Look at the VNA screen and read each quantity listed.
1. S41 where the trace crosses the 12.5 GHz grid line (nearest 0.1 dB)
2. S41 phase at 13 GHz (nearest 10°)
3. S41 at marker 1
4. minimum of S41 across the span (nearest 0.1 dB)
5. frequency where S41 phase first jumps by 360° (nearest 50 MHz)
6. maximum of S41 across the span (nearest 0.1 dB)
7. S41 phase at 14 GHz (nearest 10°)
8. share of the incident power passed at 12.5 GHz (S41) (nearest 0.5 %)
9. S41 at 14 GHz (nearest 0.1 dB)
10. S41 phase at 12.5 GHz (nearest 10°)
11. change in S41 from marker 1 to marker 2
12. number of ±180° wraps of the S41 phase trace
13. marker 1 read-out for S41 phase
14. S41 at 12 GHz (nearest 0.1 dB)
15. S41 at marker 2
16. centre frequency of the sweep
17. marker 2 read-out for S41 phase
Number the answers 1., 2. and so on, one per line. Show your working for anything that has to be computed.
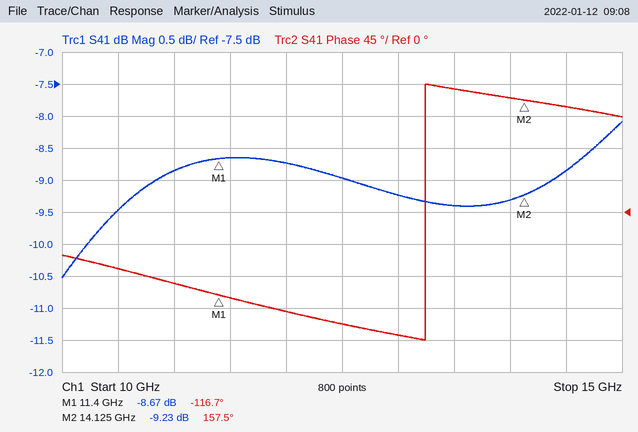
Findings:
1. -9.0 dB
2. -170°
3. -8.67 dB
4. -10.5 dB
5. 13.25 GHz
6. -8.1 dB
7. 160°
8. 10^(-9/10) ≈ 12.6 %, so 12.5 % to the nearest 0.5 %
9. -9.3 dB
10. -160°
11. -9.23 − (-8.67) = -0.56 dB
12. 1
13. -116.7°
14. -8.7 dB
15. -9.23 dB
16. 12.5 GHz
17. 157.5°
